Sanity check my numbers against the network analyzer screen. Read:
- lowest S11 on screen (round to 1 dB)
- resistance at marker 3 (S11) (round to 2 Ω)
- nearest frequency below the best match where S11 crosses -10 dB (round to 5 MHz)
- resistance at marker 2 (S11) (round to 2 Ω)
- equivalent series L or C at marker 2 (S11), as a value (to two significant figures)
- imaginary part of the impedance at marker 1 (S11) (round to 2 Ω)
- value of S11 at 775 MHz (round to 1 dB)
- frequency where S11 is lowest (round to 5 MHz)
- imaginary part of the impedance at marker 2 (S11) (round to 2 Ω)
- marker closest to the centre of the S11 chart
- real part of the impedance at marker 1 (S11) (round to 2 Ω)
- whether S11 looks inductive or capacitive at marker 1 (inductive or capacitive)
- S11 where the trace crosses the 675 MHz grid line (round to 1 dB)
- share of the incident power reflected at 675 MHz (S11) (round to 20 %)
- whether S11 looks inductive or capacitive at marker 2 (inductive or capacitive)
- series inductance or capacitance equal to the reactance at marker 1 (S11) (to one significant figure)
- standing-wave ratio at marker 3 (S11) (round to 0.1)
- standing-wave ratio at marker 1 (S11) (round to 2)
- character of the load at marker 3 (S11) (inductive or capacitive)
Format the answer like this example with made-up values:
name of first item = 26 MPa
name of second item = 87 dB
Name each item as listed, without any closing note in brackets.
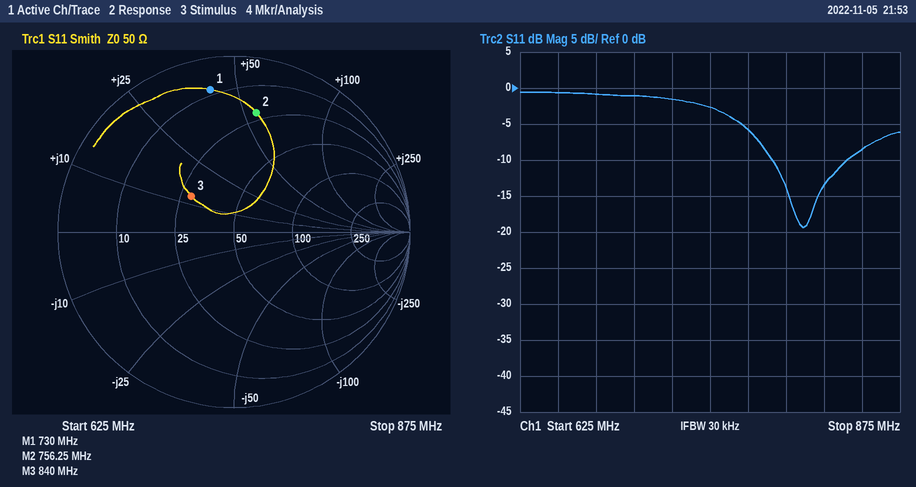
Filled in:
lowest S11 on screen = -19 dB
resistance at marker 3 (S11) = 28 Ω
nearest frequency below the best match where S11 crosses -10 dB = 790 MHz
resistance at marker 2 (S11) = 22 Ω
equivalent series L or C at marker 2 (S11), as a value = 12 nH
imaginary part of the impedance at marker 1 (S11) = +42 Ω
value of S11 at 775 MHz = -6 dB
frequency where S11 is lowest = 810 MHz
imaginary part of the impedance at marker 2 (S11) = +56 Ω
marker closest to the centre of the S11 chart = marker 3
real part of the impedance at marker 1 (S11) = 8 Ω
whether S11 looks inductive or capacitive at marker 1 = inductive
S11 where the trace crosses the 675 MHz grid line = -1 dB
share of the incident power reflected at 675 MHz (S11) = 80 %
whether S11 looks inductive or capacitive at marker 2 = inductive
series inductance or capacitance equal to the reactance at marker 1 (S11) = 9 nH
standing-wave ratio at marker 3 (S11) = 1.9
standing-wave ratio at marker 1 (S11) = 10
character of the load at marker 3 (S11) = inductive
